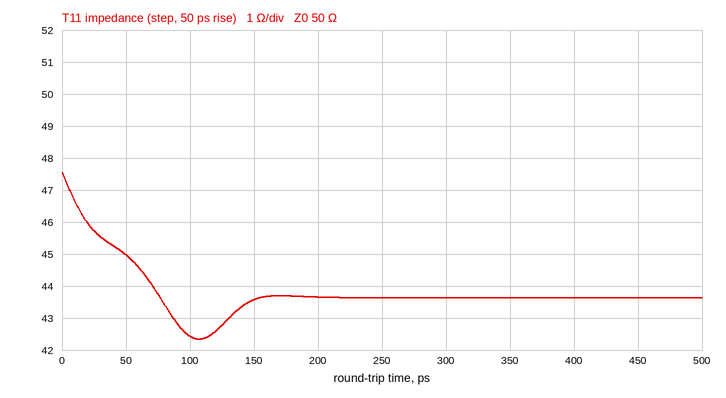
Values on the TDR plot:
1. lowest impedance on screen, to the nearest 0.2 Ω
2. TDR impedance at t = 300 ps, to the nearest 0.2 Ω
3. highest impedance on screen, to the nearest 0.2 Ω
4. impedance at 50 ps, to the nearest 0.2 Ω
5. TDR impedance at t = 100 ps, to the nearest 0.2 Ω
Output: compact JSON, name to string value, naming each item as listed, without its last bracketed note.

{"lowest impedance on screen, to the nearest 0.2 Ω": "42.4 Ω", "TDR impedance at t = 300 ps, to the nearest 0.2 Ω": "43.6 Ω", "highest impedance on screen, to the nearest 0.2 Ω": "47.6 Ω", "impedance at 50 ps, to the nearest 0.2 Ω": "45.0 Ω", "TDR impedance at t = 100 ps, to the nearest 0.2 Ω": "42.4 Ω"}
